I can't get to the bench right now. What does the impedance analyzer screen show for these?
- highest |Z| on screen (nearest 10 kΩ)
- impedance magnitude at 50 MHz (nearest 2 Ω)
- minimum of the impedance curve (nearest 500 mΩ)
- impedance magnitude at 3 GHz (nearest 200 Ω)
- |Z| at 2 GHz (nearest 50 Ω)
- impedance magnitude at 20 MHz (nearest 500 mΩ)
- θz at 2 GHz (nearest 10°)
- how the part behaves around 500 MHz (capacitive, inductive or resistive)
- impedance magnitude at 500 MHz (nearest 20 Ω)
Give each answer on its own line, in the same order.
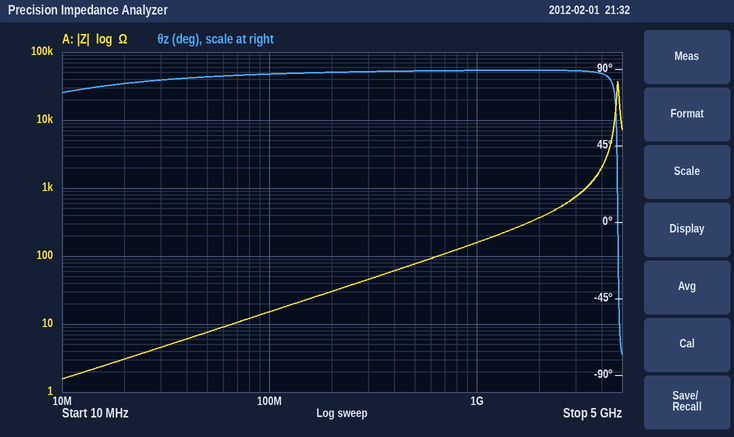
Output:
40 kΩ
8 Ω
1.5 Ω
800 Ω
350 Ω
3.0 Ω
90°
inductive
80 Ω
